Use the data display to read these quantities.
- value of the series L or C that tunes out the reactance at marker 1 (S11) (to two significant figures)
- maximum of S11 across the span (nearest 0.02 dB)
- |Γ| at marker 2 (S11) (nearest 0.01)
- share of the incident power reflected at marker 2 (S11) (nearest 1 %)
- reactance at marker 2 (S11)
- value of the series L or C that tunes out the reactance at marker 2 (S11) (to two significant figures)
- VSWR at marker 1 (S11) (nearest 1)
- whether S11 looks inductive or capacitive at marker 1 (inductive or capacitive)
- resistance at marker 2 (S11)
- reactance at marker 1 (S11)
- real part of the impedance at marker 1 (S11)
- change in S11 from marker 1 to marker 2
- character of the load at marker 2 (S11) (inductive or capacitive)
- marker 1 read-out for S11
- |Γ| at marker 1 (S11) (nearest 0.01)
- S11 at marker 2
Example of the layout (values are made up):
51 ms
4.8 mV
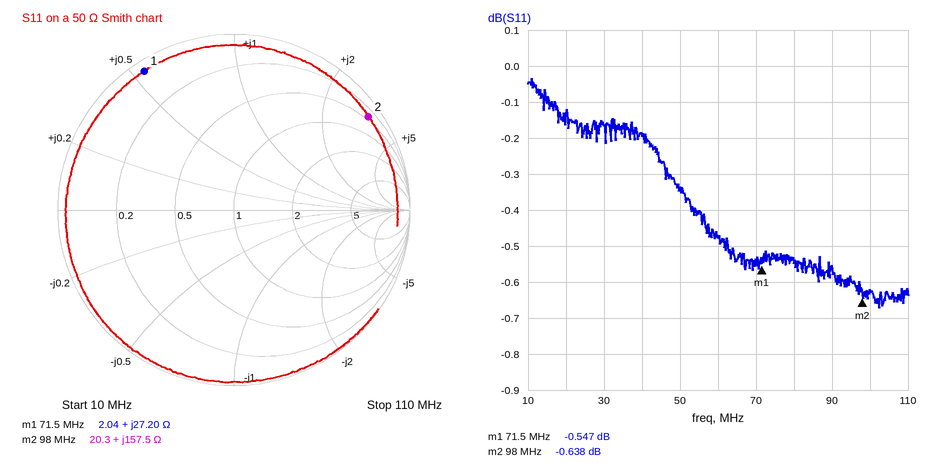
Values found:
82 pF
-0.04 dB
0.93
86 %
+157.5 Ω
10 pF
32
inductive
20.3 Ω
+27.20 Ω
2.04 Ω
-0.091 dB
inductive
-0.547 dB
0.94
-0.638 dB
